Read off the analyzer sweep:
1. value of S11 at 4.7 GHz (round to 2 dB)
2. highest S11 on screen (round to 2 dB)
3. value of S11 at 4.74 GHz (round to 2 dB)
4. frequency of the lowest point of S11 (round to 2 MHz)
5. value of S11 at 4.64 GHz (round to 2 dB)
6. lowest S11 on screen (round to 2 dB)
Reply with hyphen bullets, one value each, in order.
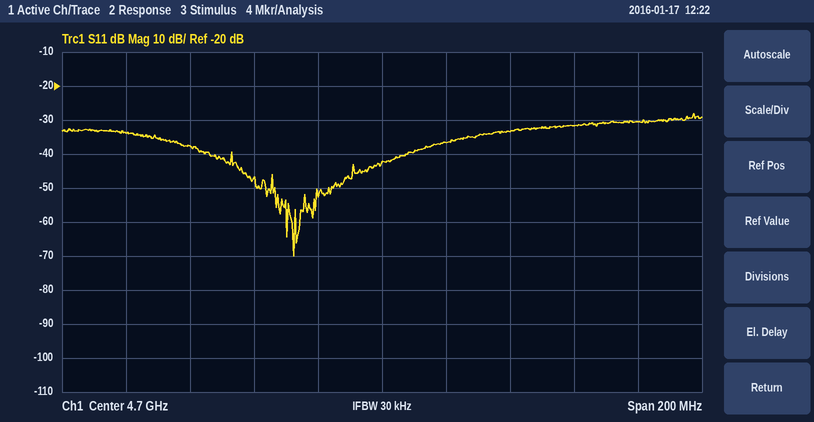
- -42 dB
- -28 dB
- -34 dB
- 4.672 GHz
- -38 dB
- -70 dB
